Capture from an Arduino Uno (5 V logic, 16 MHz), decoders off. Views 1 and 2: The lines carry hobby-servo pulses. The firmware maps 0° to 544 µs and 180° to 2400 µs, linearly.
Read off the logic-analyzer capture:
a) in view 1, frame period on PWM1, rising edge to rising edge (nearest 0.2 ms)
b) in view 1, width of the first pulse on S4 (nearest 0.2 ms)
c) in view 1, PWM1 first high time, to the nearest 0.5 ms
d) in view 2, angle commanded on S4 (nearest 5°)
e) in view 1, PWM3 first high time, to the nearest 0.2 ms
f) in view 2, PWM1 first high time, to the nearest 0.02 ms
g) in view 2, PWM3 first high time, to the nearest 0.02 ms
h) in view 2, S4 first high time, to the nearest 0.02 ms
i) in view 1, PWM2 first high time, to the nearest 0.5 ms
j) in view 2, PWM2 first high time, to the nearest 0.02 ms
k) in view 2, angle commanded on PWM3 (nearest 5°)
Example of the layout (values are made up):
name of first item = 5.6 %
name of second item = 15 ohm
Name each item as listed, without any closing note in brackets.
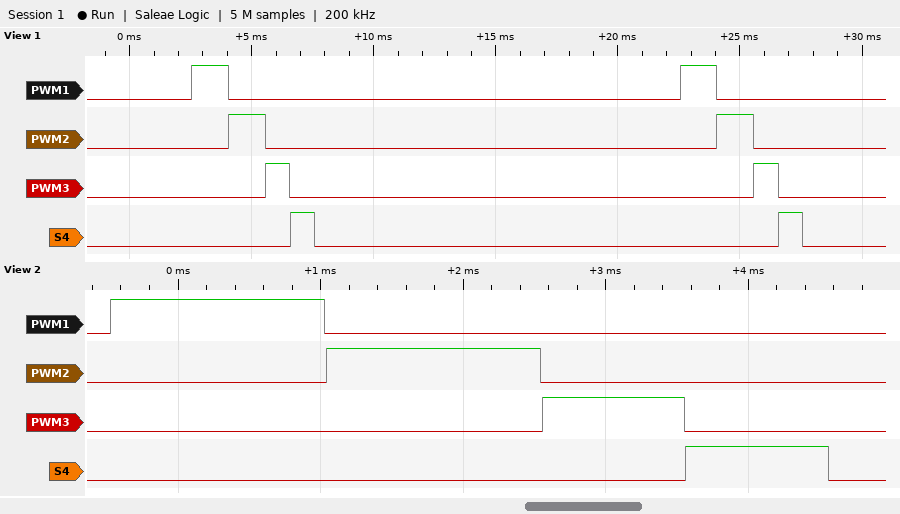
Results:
in view 1, frame period on PWM1, rising edge to rising edge = 20.0 ms
in view 1, width of the first pulse on S4 = 1.0 ms
in view 1, PWM1 first high time, to the nearest 0.5 ms = 1.5 ms
in view 2, angle commanded on S4 = 45°
in view 1, PWM3 first high time, to the nearest 0.2 ms = 1.0 ms
in view 2, PWM1 first high time, to the nearest 0.02 ms = 1.50 ms
in view 2, PWM3 first high time, to the nearest 0.02 ms = 1.00 ms
in view 2, S4 first high time, to the nearest 0.02 ms = 1.00 ms
in view 1, PWM2 first high time, to the nearest 0.5 ms = 1.5 ms
in view 2, PWM2 first high time, to the nearest 0.02 ms = 1.50 ms
in view 2, angle commanded on PWM3 = 45°
